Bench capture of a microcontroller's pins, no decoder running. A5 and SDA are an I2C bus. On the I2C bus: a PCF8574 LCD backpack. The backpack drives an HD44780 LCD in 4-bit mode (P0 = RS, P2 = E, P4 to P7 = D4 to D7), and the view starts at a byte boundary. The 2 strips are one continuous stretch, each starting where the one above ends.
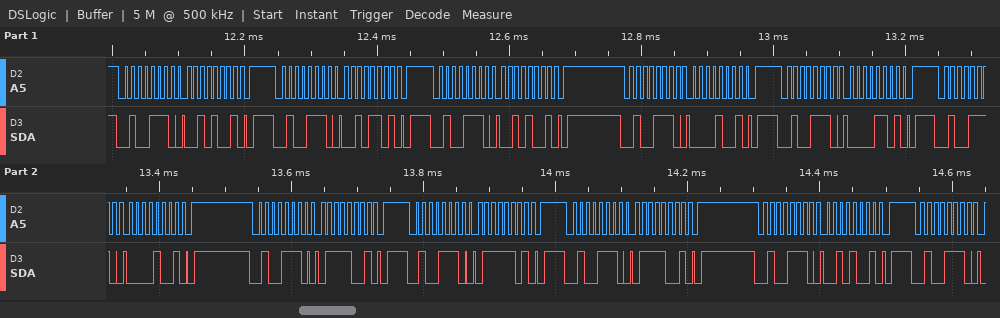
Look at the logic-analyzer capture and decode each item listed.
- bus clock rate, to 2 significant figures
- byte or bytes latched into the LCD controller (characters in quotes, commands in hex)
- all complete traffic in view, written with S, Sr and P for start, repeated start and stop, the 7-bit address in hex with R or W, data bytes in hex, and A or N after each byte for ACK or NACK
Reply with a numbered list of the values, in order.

1. 100 kHz
2. ' '
3. S 27W A 29 A P S 27W A 2D A P S 27W A 29 A P S 27W A 09 A P S 27W A 0D A P S 27W A 09 A P S 27W A 79 A P S 27W A 7D A P S 27W A 79 A P S 27W A 29 A P S 27W A
